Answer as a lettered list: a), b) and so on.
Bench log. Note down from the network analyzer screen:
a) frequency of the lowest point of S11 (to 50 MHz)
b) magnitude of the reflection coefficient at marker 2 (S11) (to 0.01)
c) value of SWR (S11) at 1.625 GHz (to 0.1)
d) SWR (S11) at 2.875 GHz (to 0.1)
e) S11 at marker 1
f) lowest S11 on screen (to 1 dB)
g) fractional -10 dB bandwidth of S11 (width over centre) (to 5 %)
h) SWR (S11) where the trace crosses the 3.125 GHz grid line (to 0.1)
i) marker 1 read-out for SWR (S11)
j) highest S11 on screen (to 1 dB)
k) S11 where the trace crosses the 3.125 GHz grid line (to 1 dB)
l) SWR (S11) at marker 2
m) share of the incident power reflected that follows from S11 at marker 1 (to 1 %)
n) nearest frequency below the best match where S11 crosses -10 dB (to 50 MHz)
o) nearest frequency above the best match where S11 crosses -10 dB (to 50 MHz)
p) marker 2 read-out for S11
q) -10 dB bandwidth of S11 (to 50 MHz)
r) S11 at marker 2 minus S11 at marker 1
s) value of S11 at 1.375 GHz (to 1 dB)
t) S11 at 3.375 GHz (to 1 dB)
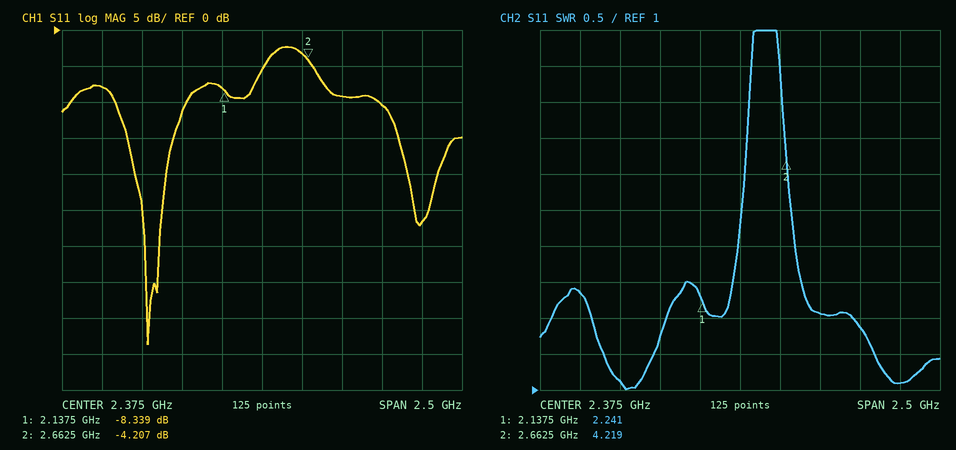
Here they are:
a) 1.65 GHz
b) 0.62
c) 1.1
d) 2.1
e) -8.339 dB
f) -44 dB
g) 25 %
h) 1.9
i) 2.241
j) -2 dB
k) -10 dB
l) 4.219
m) 15 %
n) 1.45 GHz
o) 1.90 GHz
p) -4.207 dB
q) 450 MHz
r) 4.132 dB
s) -8 dB
t) -27 dB
